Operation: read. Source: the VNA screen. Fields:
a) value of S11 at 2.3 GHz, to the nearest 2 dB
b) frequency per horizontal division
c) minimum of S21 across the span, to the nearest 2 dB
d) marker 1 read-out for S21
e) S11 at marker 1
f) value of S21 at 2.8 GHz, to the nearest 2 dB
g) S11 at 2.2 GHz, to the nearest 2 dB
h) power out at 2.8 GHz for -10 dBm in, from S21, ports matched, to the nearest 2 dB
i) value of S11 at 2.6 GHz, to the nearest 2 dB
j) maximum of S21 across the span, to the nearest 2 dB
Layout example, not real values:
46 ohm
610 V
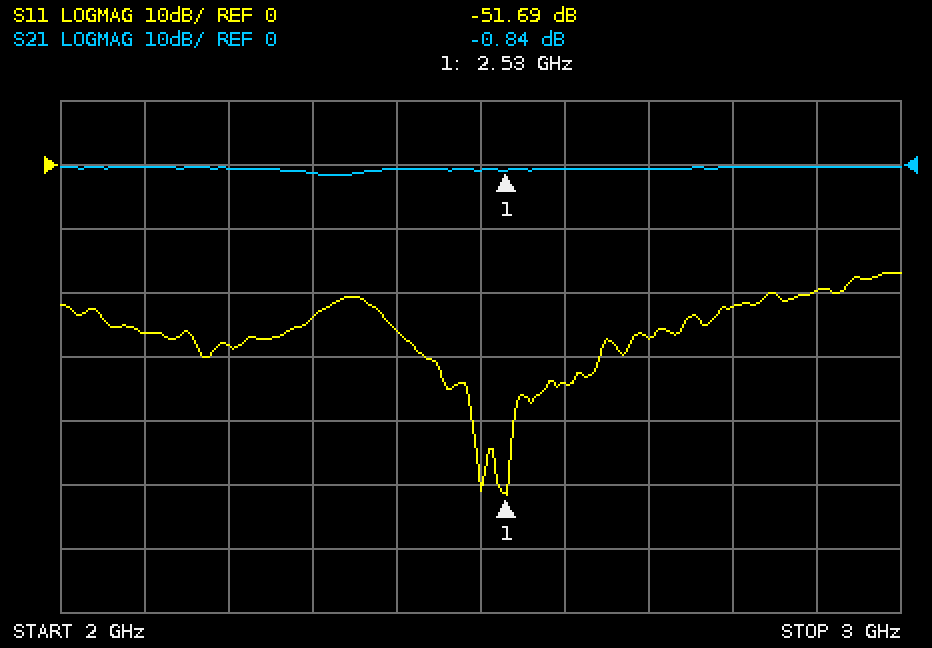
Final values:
-24 dB
100 MHz
-2 dB
-0.84 dB
-51.69 dB
0 dB
-28 dB
-10 dBm
-34 dB
0 dB
